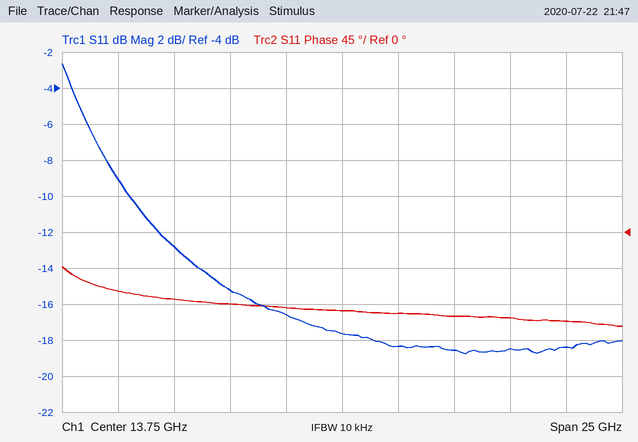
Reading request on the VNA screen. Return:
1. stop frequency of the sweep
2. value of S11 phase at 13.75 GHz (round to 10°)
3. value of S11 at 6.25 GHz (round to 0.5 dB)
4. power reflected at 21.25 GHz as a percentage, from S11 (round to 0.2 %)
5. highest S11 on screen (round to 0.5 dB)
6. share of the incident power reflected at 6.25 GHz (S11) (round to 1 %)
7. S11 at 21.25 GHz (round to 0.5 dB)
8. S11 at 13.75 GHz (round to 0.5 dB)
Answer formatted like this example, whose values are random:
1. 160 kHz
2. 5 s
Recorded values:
1. 26.25 GHz
2. -100°
3. -13.0 dB
4. 1.4 %
5. -2.5 dB
6. 5 %
7. -18.5 dB
8. -17.5 dB
